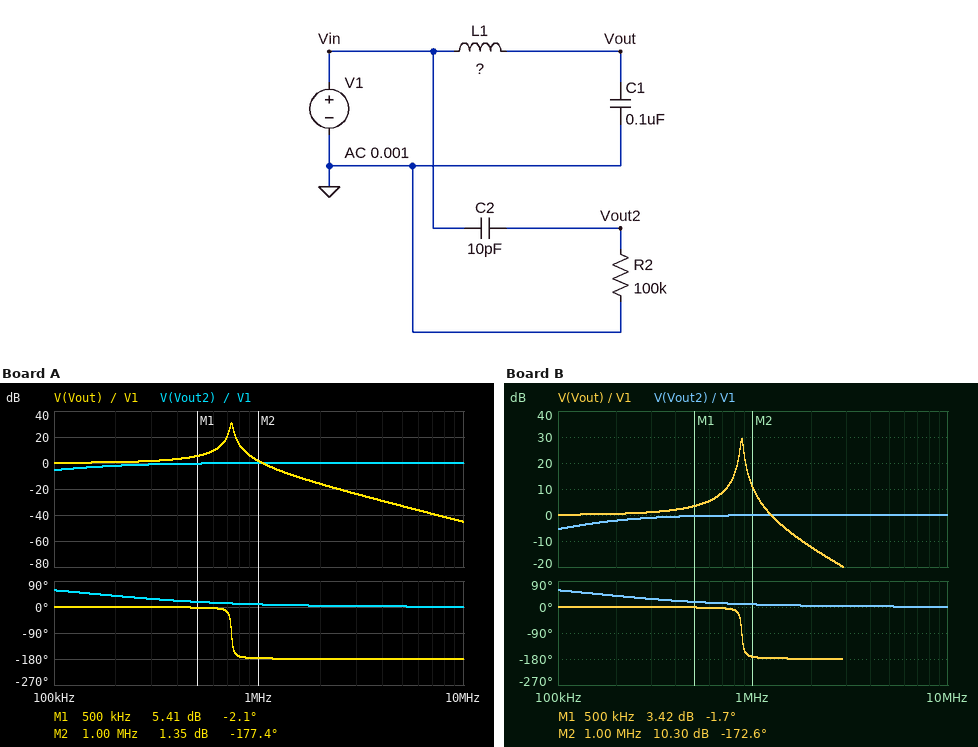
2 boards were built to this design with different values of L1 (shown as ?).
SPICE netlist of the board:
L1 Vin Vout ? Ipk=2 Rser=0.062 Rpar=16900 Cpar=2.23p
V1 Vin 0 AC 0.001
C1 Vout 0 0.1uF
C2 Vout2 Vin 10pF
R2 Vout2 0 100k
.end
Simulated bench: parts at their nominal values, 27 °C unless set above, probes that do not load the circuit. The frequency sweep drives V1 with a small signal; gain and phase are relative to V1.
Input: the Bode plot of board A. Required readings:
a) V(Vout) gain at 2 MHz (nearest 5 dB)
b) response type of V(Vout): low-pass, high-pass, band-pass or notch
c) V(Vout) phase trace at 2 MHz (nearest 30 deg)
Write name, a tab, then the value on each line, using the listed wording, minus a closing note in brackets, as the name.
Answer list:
V(Vout) gain at 2 MHz	-15 dB
response type of V(Vout): low-pass, high-pass, band-pass or notch	band-pass
V(Vout) phase trace at 2 MHz	-180 deg
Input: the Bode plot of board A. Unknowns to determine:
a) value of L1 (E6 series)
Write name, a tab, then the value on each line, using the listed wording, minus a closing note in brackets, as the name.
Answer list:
value of L1	470 nH
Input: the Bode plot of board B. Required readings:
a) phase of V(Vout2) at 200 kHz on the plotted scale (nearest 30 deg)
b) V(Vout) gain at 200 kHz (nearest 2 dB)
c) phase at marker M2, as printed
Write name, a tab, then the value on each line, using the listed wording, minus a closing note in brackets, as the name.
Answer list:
phase of V(Vout2) at 200 kHz on the plotted scale	30 deg
V(Vout) gain at 200 kHz	0 dB
phase at marker M2, as printed	-172.6 deg
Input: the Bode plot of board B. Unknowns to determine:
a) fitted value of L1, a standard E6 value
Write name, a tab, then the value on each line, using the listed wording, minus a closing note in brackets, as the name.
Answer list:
fitted value of L1, a standard E6 value	330 nH
